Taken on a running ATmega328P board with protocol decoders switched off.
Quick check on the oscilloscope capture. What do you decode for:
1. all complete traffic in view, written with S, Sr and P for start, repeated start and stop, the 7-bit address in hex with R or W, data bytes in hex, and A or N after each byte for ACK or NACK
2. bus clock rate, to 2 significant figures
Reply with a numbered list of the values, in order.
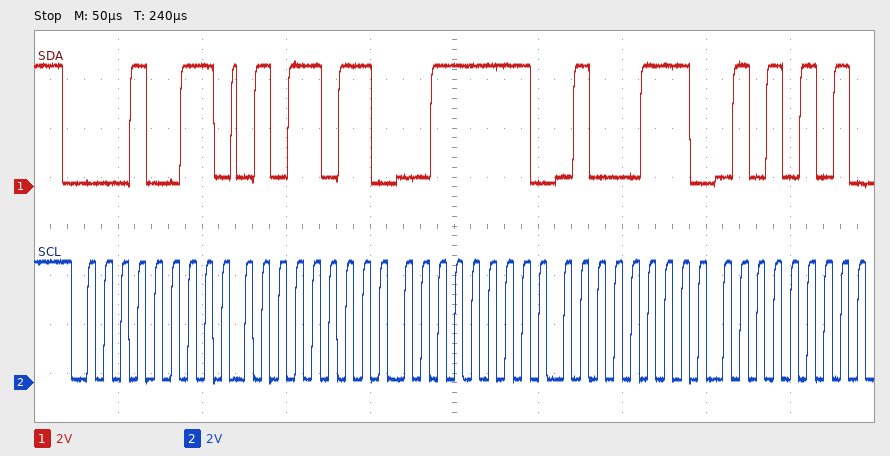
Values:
1. S 09R A 5B A 3F A 47 A 55 A
2. 100 kHz
